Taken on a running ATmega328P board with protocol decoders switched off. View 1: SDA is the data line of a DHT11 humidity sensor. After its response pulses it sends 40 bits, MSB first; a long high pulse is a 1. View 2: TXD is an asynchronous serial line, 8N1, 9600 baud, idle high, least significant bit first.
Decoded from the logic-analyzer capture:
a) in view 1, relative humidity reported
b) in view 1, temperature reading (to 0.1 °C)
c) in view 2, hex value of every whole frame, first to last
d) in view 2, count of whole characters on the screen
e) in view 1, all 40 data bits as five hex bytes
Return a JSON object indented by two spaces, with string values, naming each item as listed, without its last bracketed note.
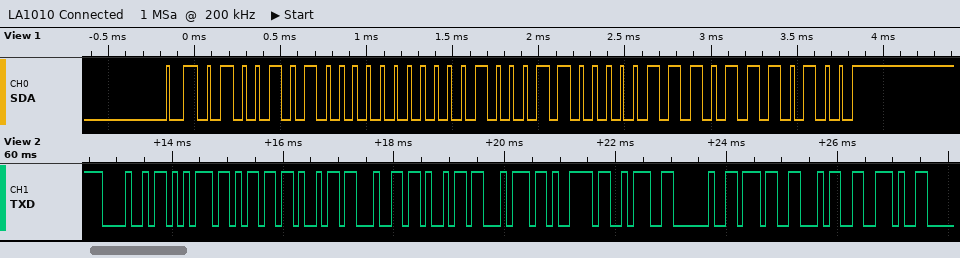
{
  "in view 1, relative humidity reported": "74 %",
  "in view 1, temperature reading": "35.7 °C",
  "in view 2, hex value of every whole frame, first to last": "48 75 6D 69 64 69 74 79 3A 20 37 34 2E",
  "in view 2, count of whole characters on the screen": "13",
  "in view 1, all 40 data bits as five hex bytes": "4A 00 23 07 74"
}
